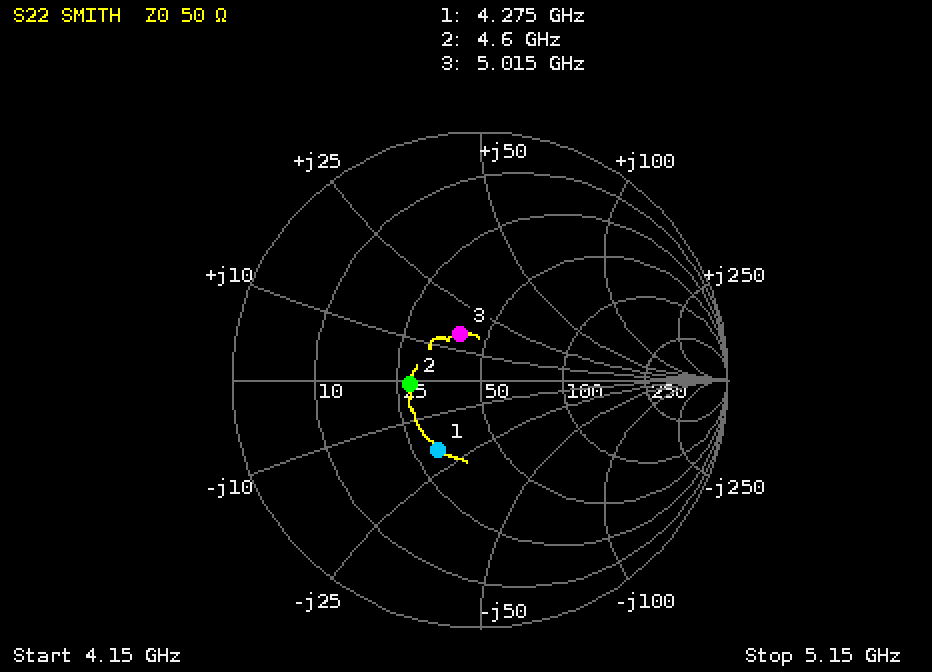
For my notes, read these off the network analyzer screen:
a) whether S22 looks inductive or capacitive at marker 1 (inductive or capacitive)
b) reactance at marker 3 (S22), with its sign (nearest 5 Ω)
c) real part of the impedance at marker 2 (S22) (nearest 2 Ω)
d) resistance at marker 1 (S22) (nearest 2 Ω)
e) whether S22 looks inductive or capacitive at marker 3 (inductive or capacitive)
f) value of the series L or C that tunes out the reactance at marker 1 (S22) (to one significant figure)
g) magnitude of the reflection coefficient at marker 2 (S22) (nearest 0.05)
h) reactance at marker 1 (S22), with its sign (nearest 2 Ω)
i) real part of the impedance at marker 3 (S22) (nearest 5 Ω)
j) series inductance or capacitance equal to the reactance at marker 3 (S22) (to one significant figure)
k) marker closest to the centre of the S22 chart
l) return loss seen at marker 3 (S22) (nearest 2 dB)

capacitive
+15 Ω
28 Ω
30 Ω
inductive
700 pH
0.30
-20 Ω
40 Ω
500 pH
marker 3
14 dB
